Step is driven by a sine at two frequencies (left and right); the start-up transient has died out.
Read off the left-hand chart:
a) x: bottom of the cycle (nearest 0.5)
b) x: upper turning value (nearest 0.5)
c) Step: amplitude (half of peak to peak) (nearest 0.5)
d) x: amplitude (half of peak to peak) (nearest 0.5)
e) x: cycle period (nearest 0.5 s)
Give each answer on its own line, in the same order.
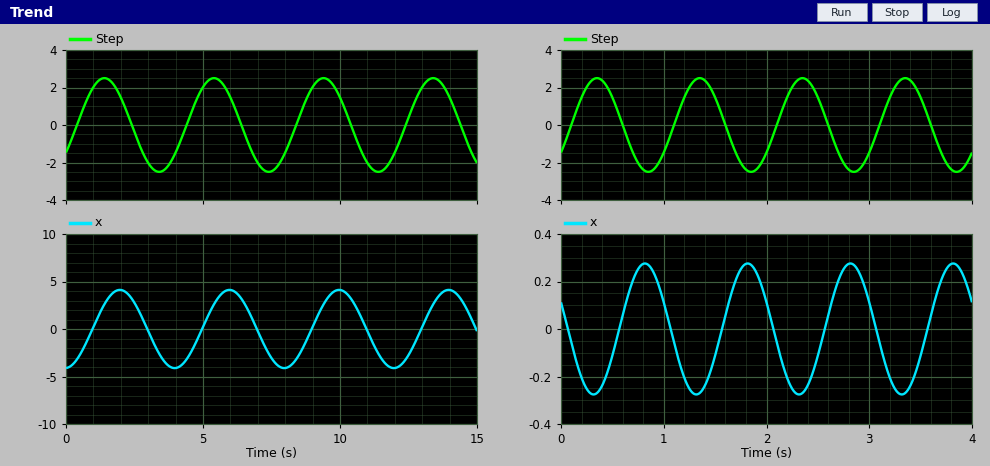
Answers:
-4.0
4.0
2.5
4.0
4.0 s
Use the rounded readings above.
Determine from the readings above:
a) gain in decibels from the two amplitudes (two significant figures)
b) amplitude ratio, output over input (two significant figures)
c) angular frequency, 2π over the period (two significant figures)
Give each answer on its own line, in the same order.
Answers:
4.1 dB
1.6
1.6 rad/s
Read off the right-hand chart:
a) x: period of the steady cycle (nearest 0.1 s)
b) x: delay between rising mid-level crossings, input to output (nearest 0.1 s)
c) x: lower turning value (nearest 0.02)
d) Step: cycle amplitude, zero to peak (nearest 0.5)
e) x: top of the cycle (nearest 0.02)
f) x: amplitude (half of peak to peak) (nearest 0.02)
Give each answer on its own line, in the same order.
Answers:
1.0 s
0.5 s
-0.28
2.5
0.28
0.28
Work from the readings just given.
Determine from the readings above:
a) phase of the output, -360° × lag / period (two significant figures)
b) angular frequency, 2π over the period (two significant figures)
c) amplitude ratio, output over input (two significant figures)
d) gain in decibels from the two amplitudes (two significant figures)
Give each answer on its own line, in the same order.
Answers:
-180°
6.3 rad/s
0.11
-19 dB
